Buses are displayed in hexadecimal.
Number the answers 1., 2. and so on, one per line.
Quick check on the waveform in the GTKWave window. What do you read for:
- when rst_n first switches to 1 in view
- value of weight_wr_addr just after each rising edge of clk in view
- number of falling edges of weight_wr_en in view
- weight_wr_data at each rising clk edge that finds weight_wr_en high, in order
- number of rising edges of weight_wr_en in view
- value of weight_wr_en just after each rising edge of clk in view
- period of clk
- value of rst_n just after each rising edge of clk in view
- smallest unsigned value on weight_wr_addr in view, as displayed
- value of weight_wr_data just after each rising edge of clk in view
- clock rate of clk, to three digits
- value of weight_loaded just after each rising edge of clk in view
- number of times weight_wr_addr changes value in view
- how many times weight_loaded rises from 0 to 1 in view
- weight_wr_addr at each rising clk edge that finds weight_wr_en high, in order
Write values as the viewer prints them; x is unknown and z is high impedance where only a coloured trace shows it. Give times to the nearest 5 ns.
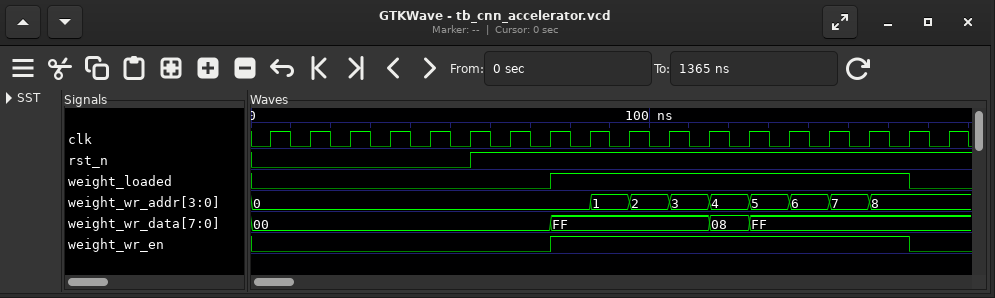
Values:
1. 55 ns
2. 0, 0, 0, 0, 0, 0, 0, 0, 1, 2, 3, 4, 5, 6, 7, 8, 8, 8
3. 1
4. FF, FF, FF, FF, 08, FF, FF, FF, FF
5. 1
6. 0 0 0 0 0 0 0 1 1 1 1 1 1 1 1 1 0 0
7. 10 ns
8. 0 0 0 0 0 1 1 1 1 1 1 1 1 1 1 1 1 1
9. 0
10. 00, 00, 00, 00, 00, 00, 00, FF, FF, FF, FF, 08, FF, FF, FF, FF, FF, FF
11. 100 MHz
12. 0 0 0 0 0 0 0 1 1 1 1 1 1 1 1 1 0 0
13. 8
14. 1
15. 0, 1, 2, 3, 4, 5, 6, 7, 8
